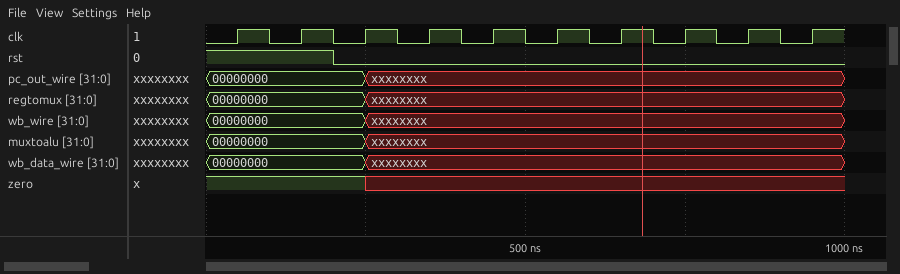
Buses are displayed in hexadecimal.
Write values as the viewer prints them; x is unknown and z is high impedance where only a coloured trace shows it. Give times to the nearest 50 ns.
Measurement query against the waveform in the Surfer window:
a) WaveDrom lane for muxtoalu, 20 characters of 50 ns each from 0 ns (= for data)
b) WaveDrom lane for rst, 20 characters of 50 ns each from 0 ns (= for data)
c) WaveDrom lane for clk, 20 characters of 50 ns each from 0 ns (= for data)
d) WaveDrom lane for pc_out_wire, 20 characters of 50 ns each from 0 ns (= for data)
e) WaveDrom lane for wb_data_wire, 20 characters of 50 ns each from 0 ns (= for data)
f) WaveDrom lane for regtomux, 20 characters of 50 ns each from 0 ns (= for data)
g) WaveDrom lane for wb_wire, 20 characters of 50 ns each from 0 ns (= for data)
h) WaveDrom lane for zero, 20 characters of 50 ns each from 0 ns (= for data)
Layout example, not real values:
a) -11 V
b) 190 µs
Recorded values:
a) {name: 'muxtoalu', wave: '=....x..............', data: '00000000'}
b) {name: 'rst', wave: '1...0...............'}
c) {name: 'clk', wave: '01010101010101010101'}
d) {name: 'pc_out_wire', wave: '=....x..............', data: '00000000'}
e) {name: 'wb_data_wire', wave: '=....x..............', data: '00000000'}
f) {name: 'regtomux', wave: '=....x..............', data: '00000000'}
g) {name: 'wb_wire', wave: '=....x..............', data: '00000000'}
h) {name: 'zero', wave: '1....x..............'}
